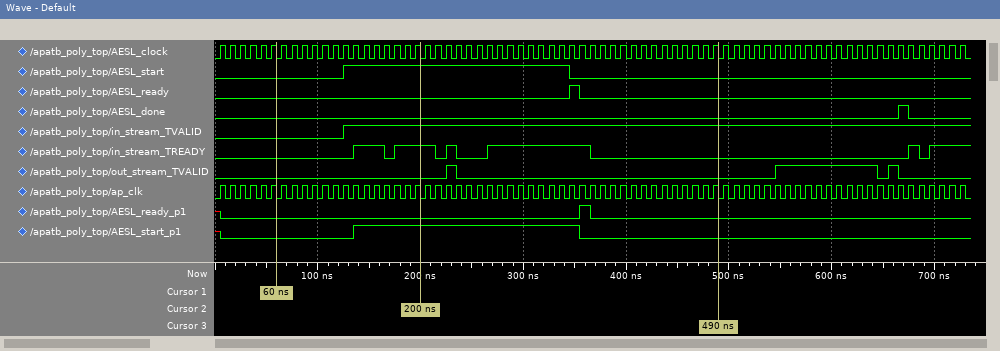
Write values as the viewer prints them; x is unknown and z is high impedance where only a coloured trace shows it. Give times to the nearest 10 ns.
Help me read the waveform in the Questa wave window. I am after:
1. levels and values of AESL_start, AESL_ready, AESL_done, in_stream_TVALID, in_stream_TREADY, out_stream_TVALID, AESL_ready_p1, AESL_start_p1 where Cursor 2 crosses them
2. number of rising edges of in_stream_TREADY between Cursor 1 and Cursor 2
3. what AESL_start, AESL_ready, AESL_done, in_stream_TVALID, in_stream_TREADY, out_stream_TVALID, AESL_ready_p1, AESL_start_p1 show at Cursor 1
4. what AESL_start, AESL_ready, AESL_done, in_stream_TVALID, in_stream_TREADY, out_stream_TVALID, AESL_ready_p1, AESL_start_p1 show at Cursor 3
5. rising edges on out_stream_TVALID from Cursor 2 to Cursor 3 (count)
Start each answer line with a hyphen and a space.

- AESL_start=1, AESL_ready=0, AESL_done=0, in_stream_TVALID=1, in_stream_TREADY=1, out_stream_TVALID=0, AESL_ready_p1=0, AESL_start_p1=1
- 2
- AESL_start=0, AESL_ready=0, AESL_done=0, in_stream_TVALID=0, in_stream_TREADY=0, out_stream_TVALID=0, AESL_ready_p1=0, AESL_start_p1=0
- AESL_start=0, AESL_ready=0, AESL_done=0, in_stream_TVALID=1, in_stream_TREADY=0, out_stream_TVALID=0, AESL_ready_p1=0, AESL_start_p1=0
- 1
